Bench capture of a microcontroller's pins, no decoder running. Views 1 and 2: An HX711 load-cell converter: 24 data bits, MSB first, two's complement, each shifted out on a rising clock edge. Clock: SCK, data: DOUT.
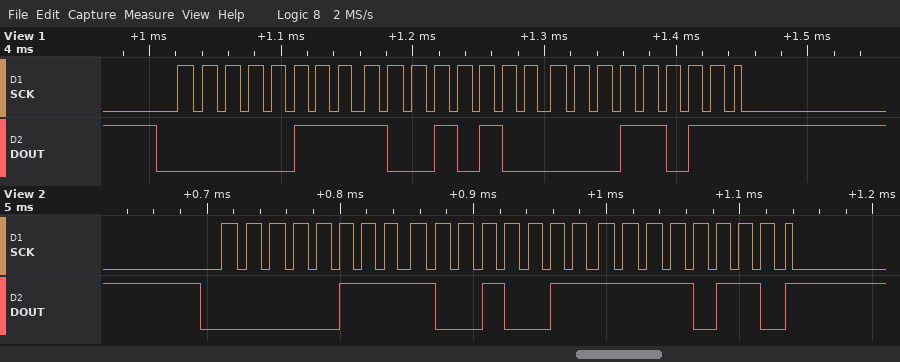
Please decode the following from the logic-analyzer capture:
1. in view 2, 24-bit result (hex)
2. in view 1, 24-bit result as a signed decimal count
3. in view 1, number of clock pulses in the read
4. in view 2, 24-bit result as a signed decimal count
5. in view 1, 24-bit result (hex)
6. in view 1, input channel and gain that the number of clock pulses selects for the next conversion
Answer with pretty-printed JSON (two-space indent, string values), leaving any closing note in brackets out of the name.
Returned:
{
  "in view 2, 24-bit result": "0x0793F6",
  "in view 1, 24-bit result as a signed decimal count": "496667",
  "in view 1, number of clock pulses in the read": "25",
  "in view 2, 24-bit result as a signed decimal count": "496630",
  "in view 1, 24-bit result": "0x07941B",
  "in view 1, input channel and gain that the number of clock pulses selects for the next conversion": "channel A, gain 128"
}
